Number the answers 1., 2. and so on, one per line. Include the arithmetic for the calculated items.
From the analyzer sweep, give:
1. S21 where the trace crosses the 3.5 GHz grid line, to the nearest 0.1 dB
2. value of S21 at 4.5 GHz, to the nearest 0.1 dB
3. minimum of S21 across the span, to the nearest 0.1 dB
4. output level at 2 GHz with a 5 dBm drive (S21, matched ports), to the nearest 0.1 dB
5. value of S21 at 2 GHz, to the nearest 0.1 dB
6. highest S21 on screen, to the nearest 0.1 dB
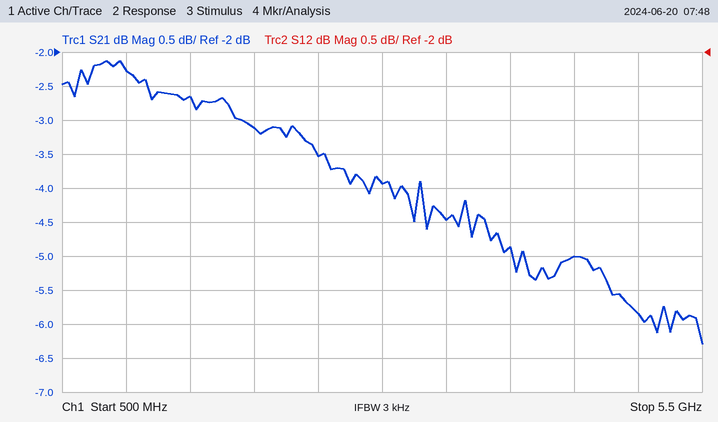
1. -4.5 dB
2. -5.0 dB
3. -6.3 dB
4. 5 dBm + (-3.1 dB) = 1.9 dBm
5. -3.1 dB
6. -2.1 dB
